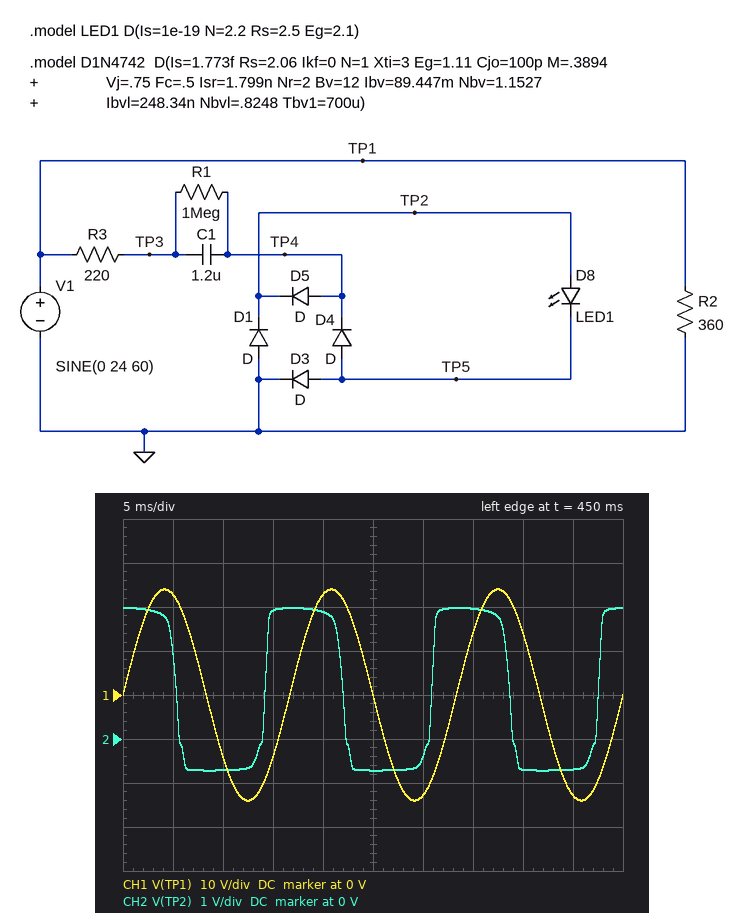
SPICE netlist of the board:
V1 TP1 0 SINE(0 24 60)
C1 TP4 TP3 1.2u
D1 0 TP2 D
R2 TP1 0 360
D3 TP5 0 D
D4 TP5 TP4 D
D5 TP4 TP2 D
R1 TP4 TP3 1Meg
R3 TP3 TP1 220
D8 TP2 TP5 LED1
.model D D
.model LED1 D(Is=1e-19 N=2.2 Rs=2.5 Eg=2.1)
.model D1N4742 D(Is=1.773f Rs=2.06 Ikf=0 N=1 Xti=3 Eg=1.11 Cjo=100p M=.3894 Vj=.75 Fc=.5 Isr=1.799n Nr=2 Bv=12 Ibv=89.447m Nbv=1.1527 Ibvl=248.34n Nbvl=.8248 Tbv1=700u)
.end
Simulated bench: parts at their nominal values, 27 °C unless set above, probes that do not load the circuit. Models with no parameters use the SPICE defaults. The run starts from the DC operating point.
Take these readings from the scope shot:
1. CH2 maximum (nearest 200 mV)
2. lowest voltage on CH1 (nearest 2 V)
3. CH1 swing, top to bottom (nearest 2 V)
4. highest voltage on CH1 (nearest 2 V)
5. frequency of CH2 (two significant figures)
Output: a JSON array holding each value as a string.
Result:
["3.0 V", "-24 V", "48 V", "24 V", "60 Hz"]
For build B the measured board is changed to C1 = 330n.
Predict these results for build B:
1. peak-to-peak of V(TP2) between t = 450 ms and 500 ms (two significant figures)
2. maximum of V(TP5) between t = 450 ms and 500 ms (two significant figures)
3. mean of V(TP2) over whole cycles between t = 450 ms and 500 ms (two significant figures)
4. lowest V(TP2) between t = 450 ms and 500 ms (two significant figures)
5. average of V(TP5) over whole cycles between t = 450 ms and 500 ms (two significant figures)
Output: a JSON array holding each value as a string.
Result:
["3.5 V", "680 mV", "960 mV", "-680 mV", "-960 mV"]
